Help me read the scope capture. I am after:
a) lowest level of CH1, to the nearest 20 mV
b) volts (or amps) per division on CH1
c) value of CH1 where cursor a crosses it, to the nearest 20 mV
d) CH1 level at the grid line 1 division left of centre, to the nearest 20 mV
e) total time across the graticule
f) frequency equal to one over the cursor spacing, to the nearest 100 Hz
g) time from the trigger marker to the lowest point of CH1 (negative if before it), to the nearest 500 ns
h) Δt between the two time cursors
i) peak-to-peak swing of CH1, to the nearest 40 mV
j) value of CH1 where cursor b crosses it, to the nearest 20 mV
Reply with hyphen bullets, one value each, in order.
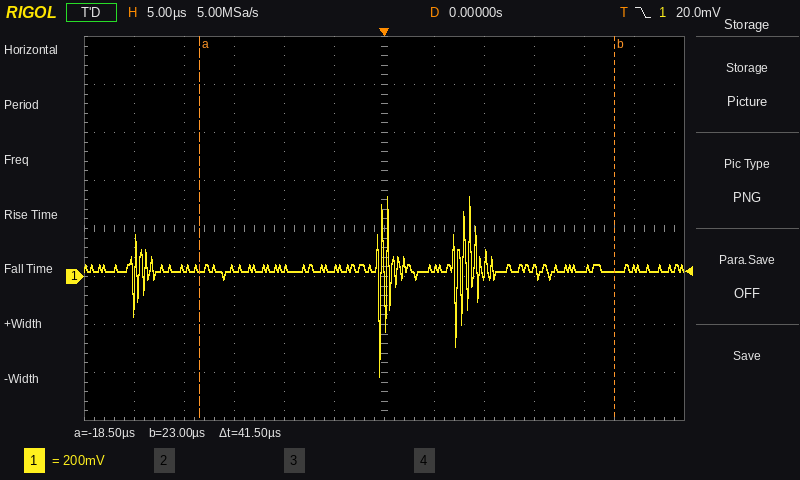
- -420 mV
- 200 mV
- 40 mV
- 40 mV
- 60 µs
- 24.1 kHz
- -500 ns
- 41.5 µs
- 760 mV
- 20 mV
